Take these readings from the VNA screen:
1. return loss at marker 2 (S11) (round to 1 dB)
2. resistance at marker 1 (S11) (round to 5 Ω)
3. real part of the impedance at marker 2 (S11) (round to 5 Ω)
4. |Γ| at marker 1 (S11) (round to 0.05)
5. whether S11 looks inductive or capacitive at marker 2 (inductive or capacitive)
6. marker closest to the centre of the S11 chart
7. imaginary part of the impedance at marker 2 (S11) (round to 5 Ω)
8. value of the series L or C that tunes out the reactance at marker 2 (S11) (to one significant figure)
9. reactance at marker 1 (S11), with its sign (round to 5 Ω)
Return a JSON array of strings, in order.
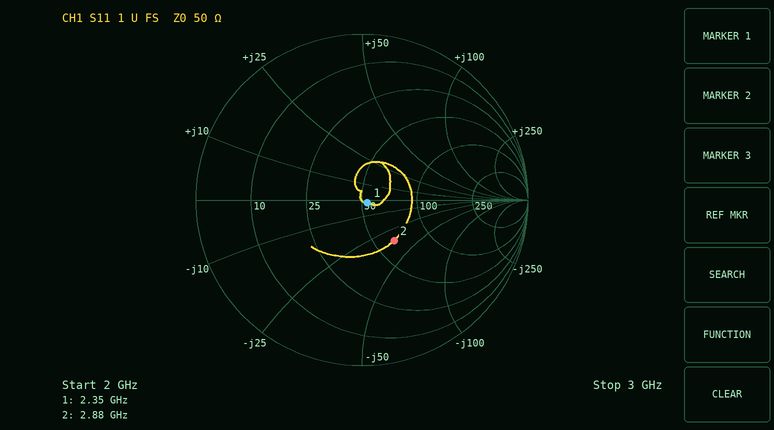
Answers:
["10 dB", "55 Ω", "65 Ω", "0.05", "capacitive", "marker 1", "-35 Ω", "2 nH", "0 Ω"]
